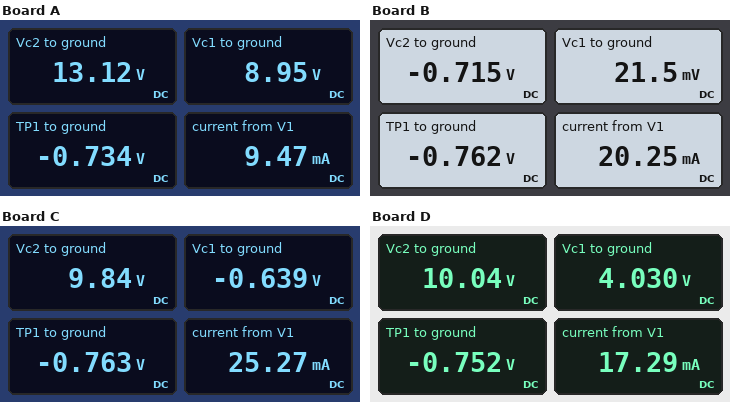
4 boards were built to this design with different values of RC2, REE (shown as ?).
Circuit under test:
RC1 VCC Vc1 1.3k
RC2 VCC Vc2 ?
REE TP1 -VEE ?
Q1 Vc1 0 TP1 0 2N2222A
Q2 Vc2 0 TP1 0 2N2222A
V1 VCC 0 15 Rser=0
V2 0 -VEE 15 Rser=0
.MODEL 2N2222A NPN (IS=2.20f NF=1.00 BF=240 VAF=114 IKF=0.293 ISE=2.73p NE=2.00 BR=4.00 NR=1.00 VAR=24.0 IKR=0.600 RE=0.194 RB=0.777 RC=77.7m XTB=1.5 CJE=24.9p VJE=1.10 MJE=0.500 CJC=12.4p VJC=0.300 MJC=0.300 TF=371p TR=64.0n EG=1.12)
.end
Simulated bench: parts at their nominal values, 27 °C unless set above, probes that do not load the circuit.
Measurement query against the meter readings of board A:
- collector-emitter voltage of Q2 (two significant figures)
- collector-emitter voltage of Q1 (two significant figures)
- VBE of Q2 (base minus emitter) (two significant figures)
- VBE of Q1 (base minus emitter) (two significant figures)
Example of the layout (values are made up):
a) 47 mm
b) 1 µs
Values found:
a) 14 V
b) 9.7 V
c) 730 mV
d) 730 mV
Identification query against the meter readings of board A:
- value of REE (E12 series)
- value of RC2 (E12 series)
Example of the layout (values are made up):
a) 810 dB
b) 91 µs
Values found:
a) 1.5 kΩ
b) 390 Ω
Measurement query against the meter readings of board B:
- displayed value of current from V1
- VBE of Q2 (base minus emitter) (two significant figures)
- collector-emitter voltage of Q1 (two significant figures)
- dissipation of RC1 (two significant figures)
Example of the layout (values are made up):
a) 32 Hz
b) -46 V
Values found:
a) 20.25 mA
b) 760 mV
c) 780 mV
d) 170 mW
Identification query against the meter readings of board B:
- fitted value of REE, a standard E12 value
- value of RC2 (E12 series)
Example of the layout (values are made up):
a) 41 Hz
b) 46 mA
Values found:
a) 680 Ω
b) 1.8 kΩ
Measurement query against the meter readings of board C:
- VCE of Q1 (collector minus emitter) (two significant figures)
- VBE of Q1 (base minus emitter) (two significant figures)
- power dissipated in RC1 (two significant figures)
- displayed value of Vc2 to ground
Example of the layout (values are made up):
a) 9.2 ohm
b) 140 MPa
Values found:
a) 120 mV
b) 760 mV
c) 190 mW
d) 9.84 V
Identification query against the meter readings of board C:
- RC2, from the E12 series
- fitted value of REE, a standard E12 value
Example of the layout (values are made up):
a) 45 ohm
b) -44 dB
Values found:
a) 390 Ω
b) 560 Ω
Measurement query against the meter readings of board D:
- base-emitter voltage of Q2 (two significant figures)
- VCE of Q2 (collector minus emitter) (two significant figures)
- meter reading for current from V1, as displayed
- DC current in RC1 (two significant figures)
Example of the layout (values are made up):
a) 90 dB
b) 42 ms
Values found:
a) 750 mV
b) 11 V
c) 17.29 mA
d) 8.4 mA
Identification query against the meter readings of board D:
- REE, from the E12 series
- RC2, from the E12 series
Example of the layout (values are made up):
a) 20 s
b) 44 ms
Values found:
a) 820 Ω
b) 560 Ω
